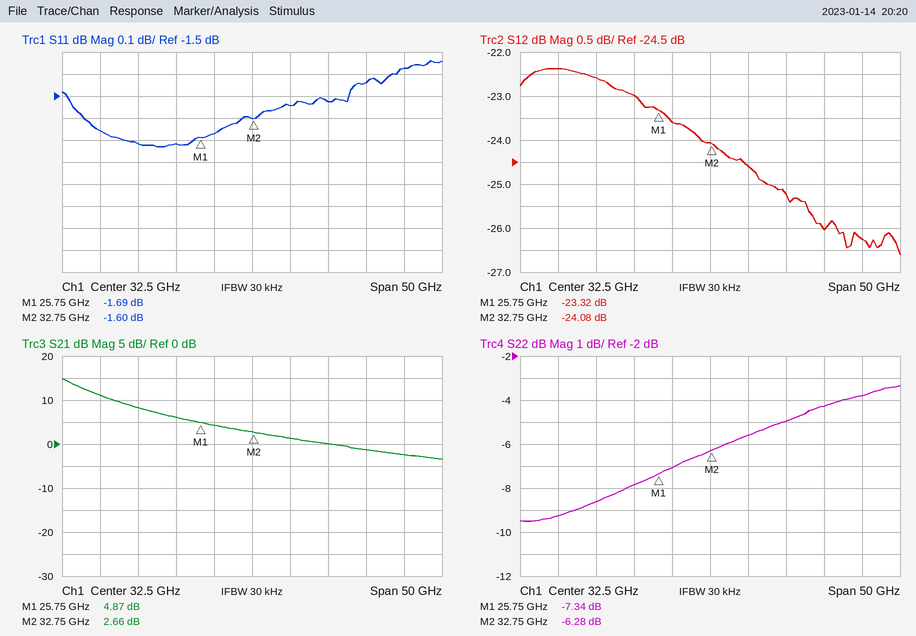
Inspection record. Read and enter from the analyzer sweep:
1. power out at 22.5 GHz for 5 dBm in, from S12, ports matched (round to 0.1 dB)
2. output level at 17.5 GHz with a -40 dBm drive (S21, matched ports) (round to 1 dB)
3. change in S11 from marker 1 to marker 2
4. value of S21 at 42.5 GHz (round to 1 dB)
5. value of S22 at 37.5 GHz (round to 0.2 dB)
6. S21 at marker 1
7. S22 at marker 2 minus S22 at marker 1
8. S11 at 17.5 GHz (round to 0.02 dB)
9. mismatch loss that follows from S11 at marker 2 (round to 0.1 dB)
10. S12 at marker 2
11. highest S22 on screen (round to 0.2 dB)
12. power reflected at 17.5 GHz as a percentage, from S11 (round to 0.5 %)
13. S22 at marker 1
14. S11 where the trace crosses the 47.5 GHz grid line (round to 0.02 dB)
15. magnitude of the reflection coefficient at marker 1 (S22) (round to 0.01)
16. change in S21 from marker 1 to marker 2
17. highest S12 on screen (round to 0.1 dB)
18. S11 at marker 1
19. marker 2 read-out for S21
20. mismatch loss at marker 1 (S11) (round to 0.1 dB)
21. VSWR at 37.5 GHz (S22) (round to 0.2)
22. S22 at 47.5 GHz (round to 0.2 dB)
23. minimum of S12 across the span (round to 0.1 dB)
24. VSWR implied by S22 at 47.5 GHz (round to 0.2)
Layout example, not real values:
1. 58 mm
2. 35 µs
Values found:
1. -18.0 dBm
2. -32 dBm
3. 0.09 dB
4. 0 dB
5. -5.6 dB
6. 4.87 dB
7. 1.06 dB
8. -1.72 dB
9. 5.1 dB
10. -24.08 dB
11. -3.4 dB
12. 67.5 %
13. -7.34 dB
14. -1.44 dB
15. 0.43
16. -2.21 dB
17. -22.4 dB
18. -1.69 dB
19. 2.66 dB
20. 4.9 dB
21. 3.2
22. -4.2 dB
23. -26.6 dB
24. 4.2
